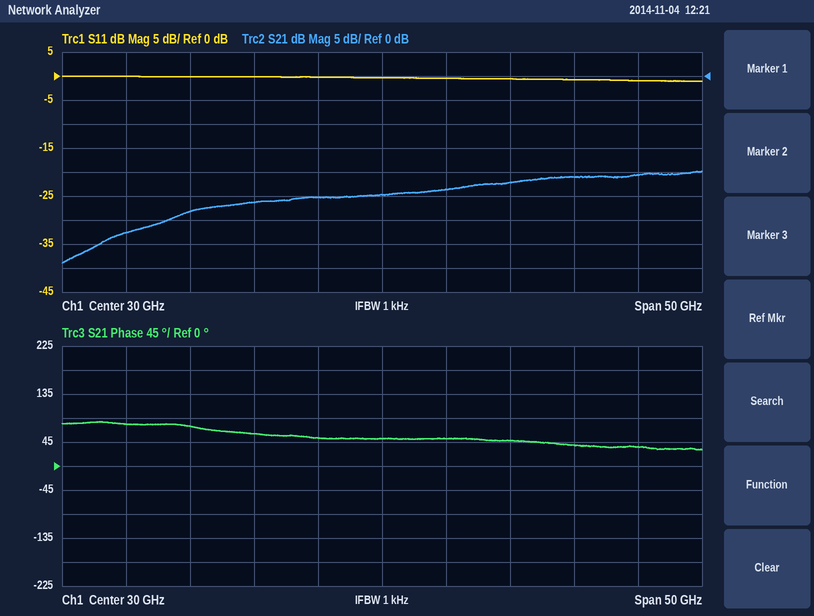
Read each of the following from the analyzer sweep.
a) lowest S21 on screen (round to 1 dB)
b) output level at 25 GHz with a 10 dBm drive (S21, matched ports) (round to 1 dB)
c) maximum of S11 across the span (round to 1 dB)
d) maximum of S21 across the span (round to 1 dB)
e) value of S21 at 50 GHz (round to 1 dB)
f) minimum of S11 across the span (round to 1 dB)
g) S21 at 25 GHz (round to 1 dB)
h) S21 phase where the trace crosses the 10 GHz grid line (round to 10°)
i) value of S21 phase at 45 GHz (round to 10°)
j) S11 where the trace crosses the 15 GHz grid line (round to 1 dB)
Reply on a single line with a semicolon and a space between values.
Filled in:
-39 dB; -15 dBm; 0 dB; -20 dB; -21 dB; -1 dB; -25 dB; 80°; 40°; 0 dB
